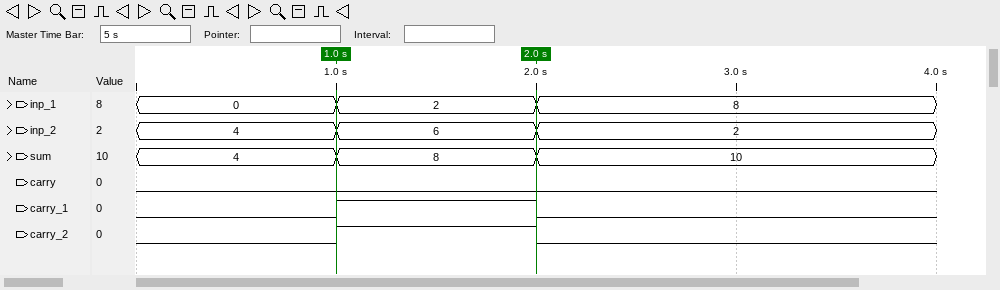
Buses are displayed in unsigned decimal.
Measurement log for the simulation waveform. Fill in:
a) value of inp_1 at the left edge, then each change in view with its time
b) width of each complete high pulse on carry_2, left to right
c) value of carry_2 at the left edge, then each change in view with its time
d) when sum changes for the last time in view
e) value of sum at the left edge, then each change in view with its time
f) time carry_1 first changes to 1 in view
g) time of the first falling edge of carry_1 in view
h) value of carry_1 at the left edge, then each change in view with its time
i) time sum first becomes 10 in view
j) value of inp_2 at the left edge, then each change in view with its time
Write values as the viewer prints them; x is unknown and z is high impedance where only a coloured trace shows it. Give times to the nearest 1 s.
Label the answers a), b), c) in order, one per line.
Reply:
a) 0, 2 at 1 s, 8 at 2 s
b) 1 s
c) 0, 1 at 1 s, 0 at 2 s
d) 2 s
e) 4, 8 at 1 s, 10 at 2 s
f) 1 s
g) 2 s
h) 0, 1 at 1 s, 0 at 2 s
i) 2 s
j) 4, 6 at 1 s, 2 at 2 s
